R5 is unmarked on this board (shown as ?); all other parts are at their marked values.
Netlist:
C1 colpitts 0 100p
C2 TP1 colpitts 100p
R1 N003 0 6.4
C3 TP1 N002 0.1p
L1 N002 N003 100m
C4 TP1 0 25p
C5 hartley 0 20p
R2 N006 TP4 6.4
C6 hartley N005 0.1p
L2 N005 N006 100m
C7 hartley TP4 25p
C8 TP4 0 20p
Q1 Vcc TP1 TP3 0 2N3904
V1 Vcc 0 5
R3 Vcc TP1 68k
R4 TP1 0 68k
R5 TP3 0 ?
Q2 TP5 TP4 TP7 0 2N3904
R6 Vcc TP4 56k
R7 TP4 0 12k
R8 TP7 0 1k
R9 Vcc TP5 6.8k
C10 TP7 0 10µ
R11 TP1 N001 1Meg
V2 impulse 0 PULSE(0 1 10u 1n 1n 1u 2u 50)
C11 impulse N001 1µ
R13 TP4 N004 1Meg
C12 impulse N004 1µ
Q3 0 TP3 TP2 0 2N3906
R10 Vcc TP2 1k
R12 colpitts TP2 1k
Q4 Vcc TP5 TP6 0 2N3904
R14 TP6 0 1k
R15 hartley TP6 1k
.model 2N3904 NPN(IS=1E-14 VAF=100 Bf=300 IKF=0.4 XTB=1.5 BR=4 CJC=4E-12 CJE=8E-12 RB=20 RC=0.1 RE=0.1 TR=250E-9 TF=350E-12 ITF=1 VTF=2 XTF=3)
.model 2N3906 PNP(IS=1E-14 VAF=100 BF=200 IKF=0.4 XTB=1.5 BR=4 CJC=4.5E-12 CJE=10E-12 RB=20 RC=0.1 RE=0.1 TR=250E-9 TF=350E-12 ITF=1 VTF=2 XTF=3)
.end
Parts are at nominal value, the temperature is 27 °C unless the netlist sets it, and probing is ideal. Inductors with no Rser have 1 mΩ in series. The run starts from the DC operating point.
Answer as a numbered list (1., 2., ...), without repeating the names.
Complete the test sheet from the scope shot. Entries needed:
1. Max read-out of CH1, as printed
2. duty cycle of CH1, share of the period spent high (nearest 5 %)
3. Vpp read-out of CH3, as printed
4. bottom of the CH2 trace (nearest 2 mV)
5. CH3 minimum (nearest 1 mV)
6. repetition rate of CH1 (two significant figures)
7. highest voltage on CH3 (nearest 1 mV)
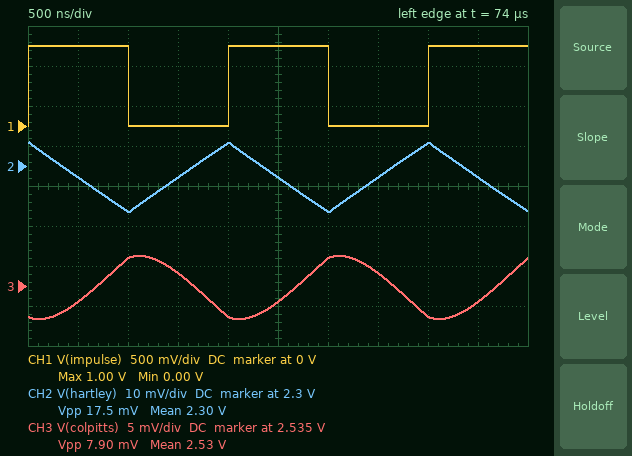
1. 1.00 V
2. 50 %
3. 7.90 mV
4. 2.288 V
5. 2.531 V
6. 500 kHz
7. 2.539 V
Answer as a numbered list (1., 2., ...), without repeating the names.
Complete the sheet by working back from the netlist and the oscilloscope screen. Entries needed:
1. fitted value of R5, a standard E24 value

1. 5.6 kΩ
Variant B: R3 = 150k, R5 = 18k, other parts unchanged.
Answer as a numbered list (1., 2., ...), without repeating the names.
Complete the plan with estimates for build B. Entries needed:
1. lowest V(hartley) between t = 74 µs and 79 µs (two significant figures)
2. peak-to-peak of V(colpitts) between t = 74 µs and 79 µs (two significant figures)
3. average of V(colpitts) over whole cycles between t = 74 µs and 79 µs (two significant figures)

1. 2.3 V
2. 7.3 mV
3. 1.7 V
